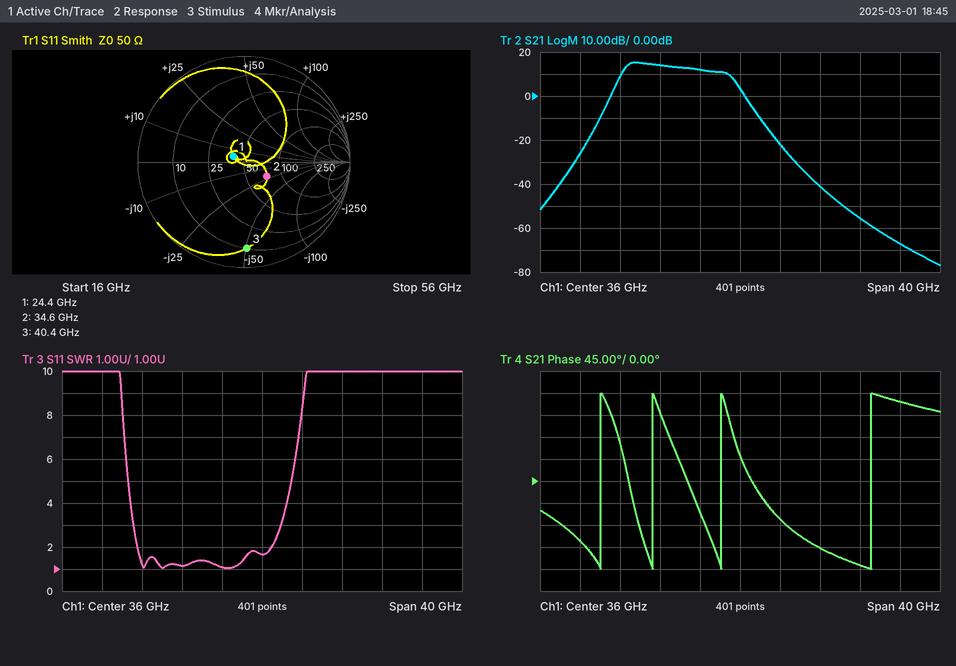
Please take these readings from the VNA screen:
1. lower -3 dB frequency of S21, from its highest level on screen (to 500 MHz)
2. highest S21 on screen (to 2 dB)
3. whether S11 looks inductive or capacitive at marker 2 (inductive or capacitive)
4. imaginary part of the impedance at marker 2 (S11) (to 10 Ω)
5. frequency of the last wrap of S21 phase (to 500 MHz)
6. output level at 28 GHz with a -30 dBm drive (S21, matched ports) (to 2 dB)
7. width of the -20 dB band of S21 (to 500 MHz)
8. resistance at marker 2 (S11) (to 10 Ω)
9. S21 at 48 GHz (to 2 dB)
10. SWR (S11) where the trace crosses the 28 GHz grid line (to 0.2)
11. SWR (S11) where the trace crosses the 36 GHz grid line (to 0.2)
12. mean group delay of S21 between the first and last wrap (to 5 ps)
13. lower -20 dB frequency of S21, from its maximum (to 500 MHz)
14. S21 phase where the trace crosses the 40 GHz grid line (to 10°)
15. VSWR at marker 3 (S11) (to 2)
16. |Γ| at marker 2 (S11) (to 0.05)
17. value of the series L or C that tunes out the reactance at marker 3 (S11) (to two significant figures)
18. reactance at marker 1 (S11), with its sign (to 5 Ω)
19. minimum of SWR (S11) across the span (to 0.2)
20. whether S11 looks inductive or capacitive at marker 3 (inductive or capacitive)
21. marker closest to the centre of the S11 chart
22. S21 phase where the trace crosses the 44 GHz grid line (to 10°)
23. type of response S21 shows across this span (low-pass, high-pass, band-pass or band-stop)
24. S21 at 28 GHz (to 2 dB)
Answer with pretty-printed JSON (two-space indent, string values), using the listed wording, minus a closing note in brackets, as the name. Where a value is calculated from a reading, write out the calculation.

{
  "lower -3 dB frequency of S21, from its highest level on screen": "24.5 GHz",
  "highest S21 on screen": "16 dB",
  "whether S11 looks inductive or capacitive at marker 2": "capacitive",
  "imaginary part of the impedance at marker 2 (S11)": "-20 Ω",
  "frequency of the last wrap of S21 phase": "49.0 GHz",
  "output level at 28 GHz with a -30 dBm drive (S21, matched ports)": "-30 dBm + (14 dB) = -16 dBm",
  "width of the -20 dB band of S21": "37.0 GHz − 22.5 GHz = 14.5 GHz",
  "resistance at marker 2 (S11)": "70 Ω",
  "S21 at 48 GHz": "-56 dB",
  "SWR (S11) where the trace crosses the 28 GHz grid line": "1.2",
  "SWR (S11) where the trace crosses the 36 GHz grid line": "1.6",
  "mean group delay of S21 between the first and last wrap": "3 cycles / (49.0 GHz − 22.0 GHz) ≈ 111 ps, so 110 ps to the nearest 5 ps",
  "lower -20 dB frequency of S21, from its maximum": "22.5 GHz",
  "S21 phase where the trace crosses the 40 GHz grid line": "-80°",
  "VSWR at marker 3 (S11)": "10",
  "|Γ| at marker 2 (S11)": "0.25",
  "value of the series L or C that tunes out the reactance at marker 3 (S11)": "L = 50 Ω/(2π × 40.4 GHz) ≈ 197 pH, so 200 pH to two significant figures",
  "reactance at marker 1 (S11), with its sign": "+5 Ω",
  "minimum of SWR (S11) across the span": "1.0",
  "whether S11 looks inductive or capacitive at marker 3": "capacitive",
  "marker closest to the centre of the S11 chart": "marker 1",
  "S21 phase where the trace crosses the 44 GHz grid line": "-140°",
  "type of response S21 shows across this span": "band-pass",
  "S21 at 28 GHz": "14 dB"
}
